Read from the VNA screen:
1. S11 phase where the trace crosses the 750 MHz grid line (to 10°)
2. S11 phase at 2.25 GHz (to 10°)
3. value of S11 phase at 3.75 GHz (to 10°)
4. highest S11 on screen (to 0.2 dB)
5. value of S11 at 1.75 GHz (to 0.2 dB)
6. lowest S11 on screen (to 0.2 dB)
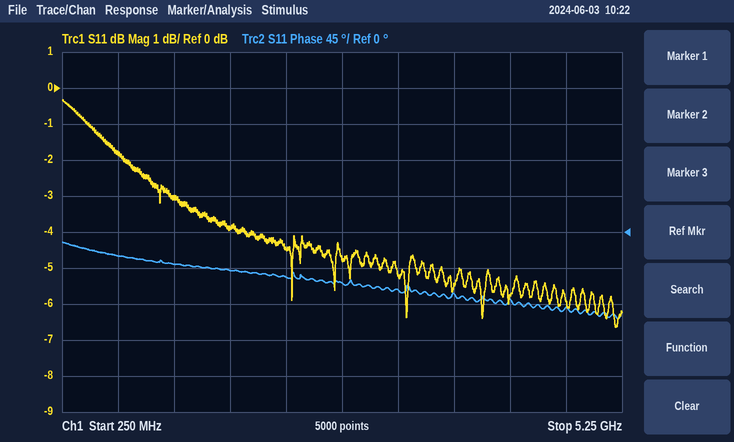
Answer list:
-30°
-60°
-80°
-0.4 dB
-3.8 dB
-6.6 dB
